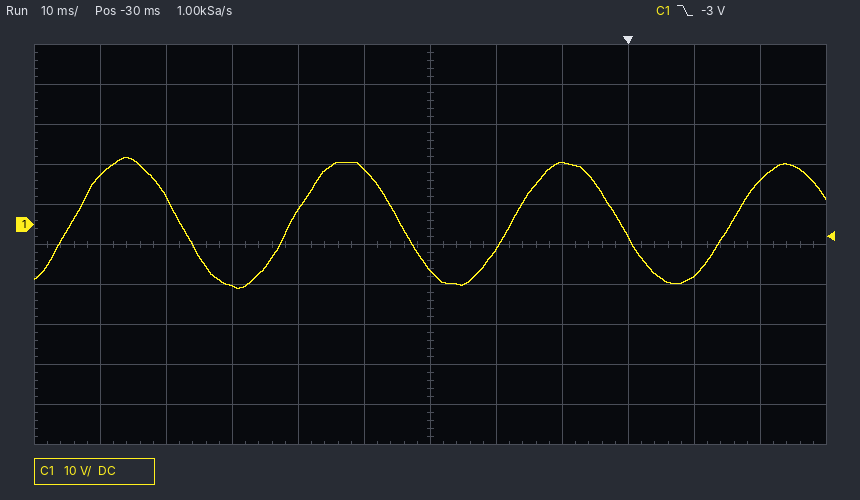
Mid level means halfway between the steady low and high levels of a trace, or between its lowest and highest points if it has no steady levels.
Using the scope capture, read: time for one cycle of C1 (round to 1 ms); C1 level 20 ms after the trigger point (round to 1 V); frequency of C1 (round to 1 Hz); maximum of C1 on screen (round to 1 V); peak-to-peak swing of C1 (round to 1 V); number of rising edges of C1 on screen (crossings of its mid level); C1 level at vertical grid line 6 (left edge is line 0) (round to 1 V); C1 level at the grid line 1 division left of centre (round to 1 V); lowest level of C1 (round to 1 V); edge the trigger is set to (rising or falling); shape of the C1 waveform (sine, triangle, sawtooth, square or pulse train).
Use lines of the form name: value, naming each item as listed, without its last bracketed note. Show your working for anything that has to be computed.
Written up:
time for one cycle of C1: 33 ms
C1 level 20 ms after the trigger point: 11 V
frequency of C1: 1 / 33 ms ≈ 30 Hz
maximum of C1 on screen: 17 V
peak-to-peak swing of C1: 17 V − (-16 V) = 33 V
number of rising edges of C1 on screen: 4
C1 level at vertical grid line 6 (left edge is line 0): -11 V
C1 level at the grid line 1 division left of centre: 14 V
lowest level of C1: -16 V
edge the trigger is set to: falling
shape of the C1 waveform: sine
